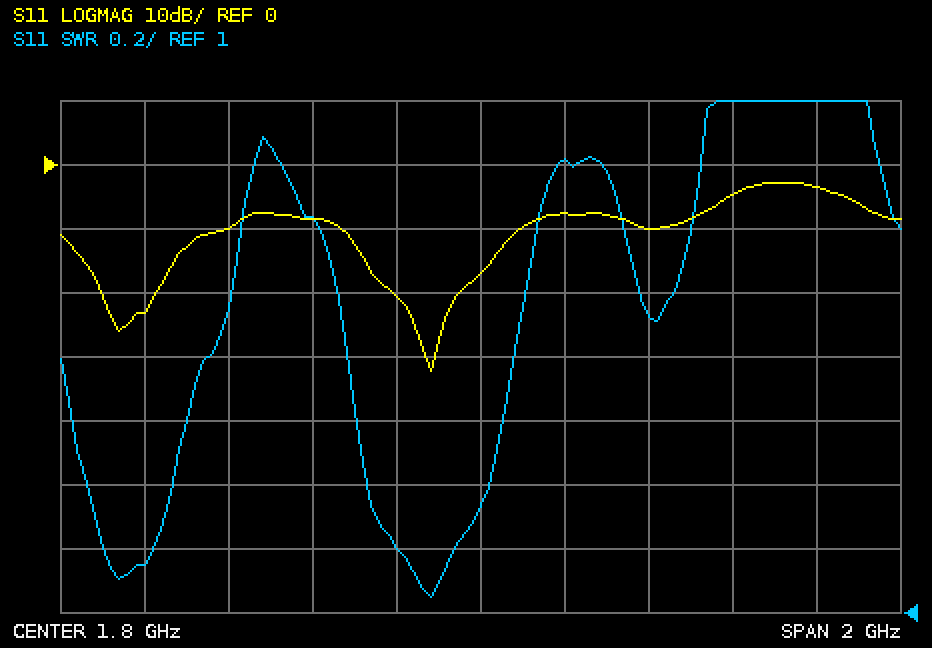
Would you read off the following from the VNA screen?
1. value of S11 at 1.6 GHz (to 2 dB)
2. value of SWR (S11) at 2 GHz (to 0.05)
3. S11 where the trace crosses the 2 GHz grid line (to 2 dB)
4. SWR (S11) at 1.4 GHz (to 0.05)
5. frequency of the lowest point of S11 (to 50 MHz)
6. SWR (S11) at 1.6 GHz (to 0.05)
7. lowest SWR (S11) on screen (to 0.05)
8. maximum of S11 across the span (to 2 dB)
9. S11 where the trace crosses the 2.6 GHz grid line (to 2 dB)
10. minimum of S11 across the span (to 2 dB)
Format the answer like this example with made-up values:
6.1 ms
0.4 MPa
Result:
-20 dB
2.40
-8 dB
2.25
1.70 GHz
1.20
1.05
-2 dB
-4 dB
-32 dB
